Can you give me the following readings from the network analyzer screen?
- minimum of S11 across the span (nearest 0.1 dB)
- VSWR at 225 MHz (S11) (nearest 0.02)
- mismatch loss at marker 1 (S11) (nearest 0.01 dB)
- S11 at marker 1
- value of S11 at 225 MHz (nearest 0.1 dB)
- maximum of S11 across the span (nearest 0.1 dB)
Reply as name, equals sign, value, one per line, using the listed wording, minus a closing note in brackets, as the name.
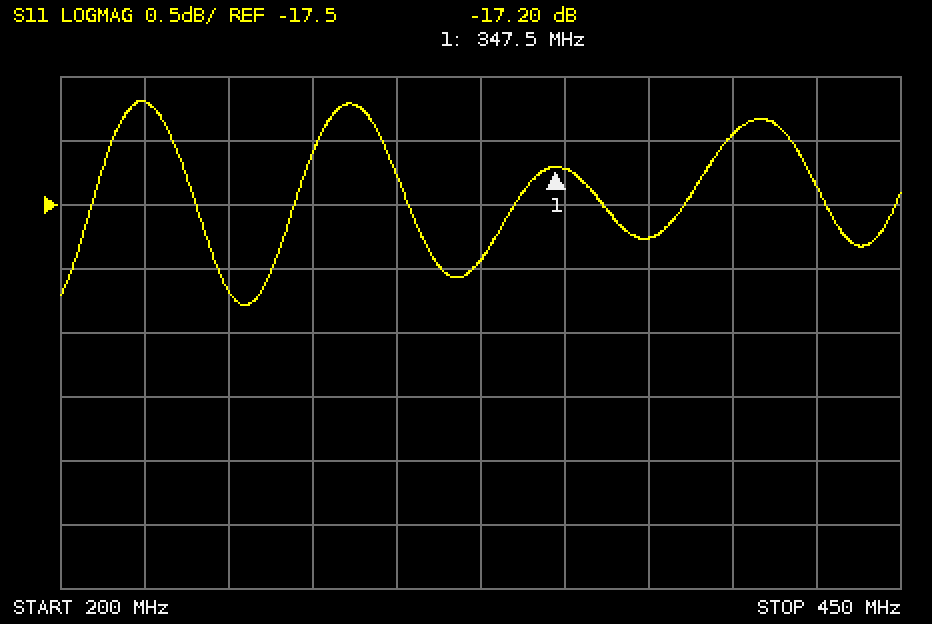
minimum of S11 across the span = -18.3 dB
VSWR at 225 MHz (S11) = 1.34
mismatch loss at marker 1 (S11) = 0.08 dB
S11 at marker 1 = -17.20 dB
value of S11 at 225 MHz = -16.7 dB
maximum of S11 across the span = -16.7 dB
